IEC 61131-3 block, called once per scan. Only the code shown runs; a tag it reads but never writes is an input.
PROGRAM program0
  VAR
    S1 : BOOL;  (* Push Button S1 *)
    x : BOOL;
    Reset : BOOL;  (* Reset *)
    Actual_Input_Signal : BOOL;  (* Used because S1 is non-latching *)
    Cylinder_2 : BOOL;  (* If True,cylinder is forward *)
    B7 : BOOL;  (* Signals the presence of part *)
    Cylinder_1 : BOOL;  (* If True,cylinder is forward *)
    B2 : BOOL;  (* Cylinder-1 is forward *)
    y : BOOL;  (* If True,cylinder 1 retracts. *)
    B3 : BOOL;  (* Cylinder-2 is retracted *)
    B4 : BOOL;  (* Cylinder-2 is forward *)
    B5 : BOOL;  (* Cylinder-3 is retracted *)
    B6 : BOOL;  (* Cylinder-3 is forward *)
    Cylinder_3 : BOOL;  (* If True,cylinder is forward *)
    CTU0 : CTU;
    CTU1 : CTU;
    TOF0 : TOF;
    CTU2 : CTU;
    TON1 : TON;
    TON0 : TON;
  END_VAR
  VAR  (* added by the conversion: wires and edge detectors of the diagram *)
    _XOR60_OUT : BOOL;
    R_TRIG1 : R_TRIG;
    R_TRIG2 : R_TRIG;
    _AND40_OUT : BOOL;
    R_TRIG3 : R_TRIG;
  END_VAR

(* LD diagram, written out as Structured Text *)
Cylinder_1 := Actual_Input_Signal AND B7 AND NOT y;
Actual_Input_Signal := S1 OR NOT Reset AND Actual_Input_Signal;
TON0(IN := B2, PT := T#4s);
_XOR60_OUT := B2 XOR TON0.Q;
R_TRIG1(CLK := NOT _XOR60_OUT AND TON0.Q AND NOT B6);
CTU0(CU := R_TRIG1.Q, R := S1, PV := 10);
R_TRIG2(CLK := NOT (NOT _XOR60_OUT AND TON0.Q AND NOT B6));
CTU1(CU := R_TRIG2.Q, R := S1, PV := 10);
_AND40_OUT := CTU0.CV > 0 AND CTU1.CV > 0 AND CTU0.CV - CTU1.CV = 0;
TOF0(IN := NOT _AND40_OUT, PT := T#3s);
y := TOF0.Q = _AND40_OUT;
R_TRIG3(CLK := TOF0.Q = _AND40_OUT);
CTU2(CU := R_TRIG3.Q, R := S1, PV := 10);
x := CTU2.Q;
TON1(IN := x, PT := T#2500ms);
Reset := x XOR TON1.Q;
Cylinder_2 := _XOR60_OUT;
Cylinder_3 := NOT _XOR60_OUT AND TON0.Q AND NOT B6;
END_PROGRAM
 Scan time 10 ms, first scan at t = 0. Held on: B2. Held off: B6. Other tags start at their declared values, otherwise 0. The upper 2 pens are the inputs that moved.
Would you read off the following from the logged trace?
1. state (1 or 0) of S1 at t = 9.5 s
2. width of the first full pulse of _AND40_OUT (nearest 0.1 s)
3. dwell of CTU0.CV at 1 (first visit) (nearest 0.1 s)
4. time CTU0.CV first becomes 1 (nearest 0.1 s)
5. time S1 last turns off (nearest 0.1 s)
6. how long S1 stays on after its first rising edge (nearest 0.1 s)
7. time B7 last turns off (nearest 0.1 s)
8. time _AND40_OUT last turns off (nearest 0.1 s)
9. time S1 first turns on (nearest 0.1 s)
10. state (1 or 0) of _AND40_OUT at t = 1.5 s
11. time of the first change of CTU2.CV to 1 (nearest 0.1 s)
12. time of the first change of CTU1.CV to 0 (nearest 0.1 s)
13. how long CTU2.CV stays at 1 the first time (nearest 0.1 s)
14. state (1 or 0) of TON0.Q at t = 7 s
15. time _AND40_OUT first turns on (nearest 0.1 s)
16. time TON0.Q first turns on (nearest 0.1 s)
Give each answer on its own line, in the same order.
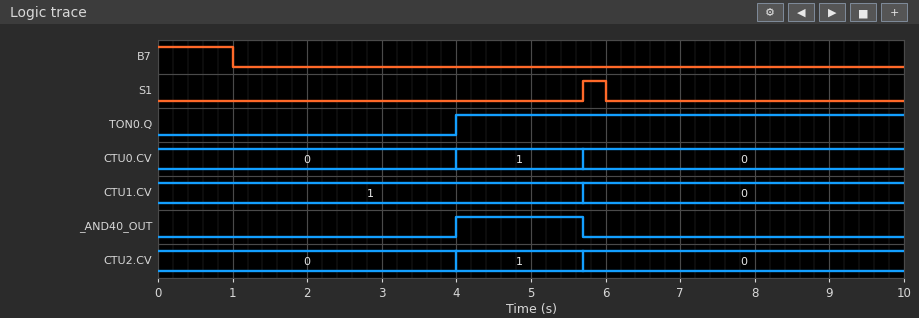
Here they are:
0
1.7 s
1.7 s
4.0 s
6.0 s
0.3 s
1.0 s
5.7 s
5.7 s
0
4.0 s
5.7 s
1.7 s
1
4.0 s
4.0 s
